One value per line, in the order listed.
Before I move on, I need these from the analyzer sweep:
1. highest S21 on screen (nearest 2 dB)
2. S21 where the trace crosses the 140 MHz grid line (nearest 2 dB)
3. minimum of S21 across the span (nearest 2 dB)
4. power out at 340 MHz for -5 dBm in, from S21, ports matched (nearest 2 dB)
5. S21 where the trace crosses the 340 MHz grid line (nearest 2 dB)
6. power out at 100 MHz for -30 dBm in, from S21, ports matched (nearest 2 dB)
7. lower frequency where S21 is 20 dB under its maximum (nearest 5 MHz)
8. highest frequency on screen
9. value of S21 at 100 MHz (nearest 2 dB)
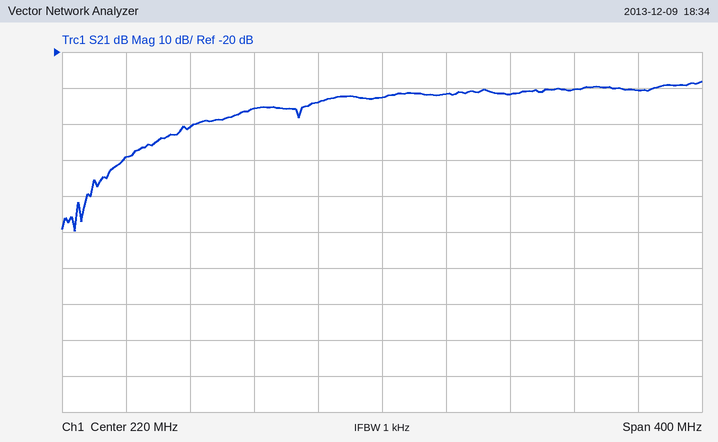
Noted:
-28 dB
-36 dB
-70 dB
-36 dBm
-30 dB
-70 dBm
65 MHz
420 MHz
-40 dB
